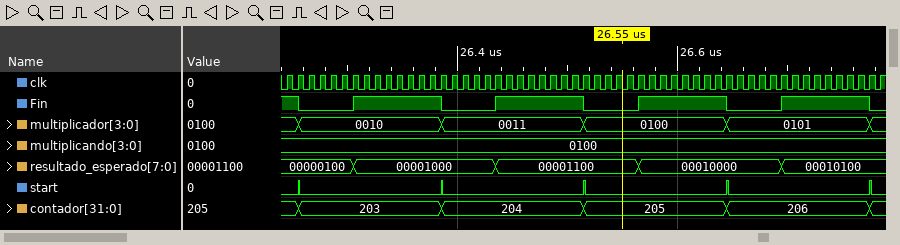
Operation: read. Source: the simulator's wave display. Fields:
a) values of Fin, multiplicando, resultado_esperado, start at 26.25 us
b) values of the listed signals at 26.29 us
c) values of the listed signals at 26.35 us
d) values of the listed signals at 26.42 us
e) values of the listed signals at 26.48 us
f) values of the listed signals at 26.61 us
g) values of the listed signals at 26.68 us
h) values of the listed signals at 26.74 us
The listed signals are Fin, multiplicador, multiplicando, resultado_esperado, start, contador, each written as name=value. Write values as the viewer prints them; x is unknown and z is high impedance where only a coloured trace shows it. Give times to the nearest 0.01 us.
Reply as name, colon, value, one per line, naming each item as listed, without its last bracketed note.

values of Fin, multiplicando, resultado_esperado, start at 26.25 us: Fin=1, multiplicando=0100, resultado_esperado=00000100, start=0
values of the listed signals at 26.29 us: Fin=0, multiplicador=0010, multiplicando=0100, resultado_esperado=00000100, start=0, contador=203
values of the listed signals at 26.35 us: Fin=1, multiplicador=0010, multiplicando=0100, resultado_esperado=00001000, start=0, contador=203
values of the listed signals at 26.42 us: Fin=0, multiplicador=0011, multiplicando=0100, resultado_esperado=00001000, start=0, contador=204
values of the listed signals at 26.48 us: Fin=1, multiplicador=0011, multiplicando=0100, resultado_esperado=00001100, start=0, contador=204
values of the listed signals at 26.61 us: Fin=1, multiplicador=0100, multiplicando=0100, resultado_esperado=00010000, start=0, contador=205
values of the listed signals at 26.68 us: Fin=0, multiplicador=0101, multiplicando=0100, resultado_esperado=00010000, start=0, contador=206
values of the listed signals at 26.74 us: Fin=1, multiplicador=0101, multiplicando=0100, resultado_esperado=00010100, start=0, contador=206
